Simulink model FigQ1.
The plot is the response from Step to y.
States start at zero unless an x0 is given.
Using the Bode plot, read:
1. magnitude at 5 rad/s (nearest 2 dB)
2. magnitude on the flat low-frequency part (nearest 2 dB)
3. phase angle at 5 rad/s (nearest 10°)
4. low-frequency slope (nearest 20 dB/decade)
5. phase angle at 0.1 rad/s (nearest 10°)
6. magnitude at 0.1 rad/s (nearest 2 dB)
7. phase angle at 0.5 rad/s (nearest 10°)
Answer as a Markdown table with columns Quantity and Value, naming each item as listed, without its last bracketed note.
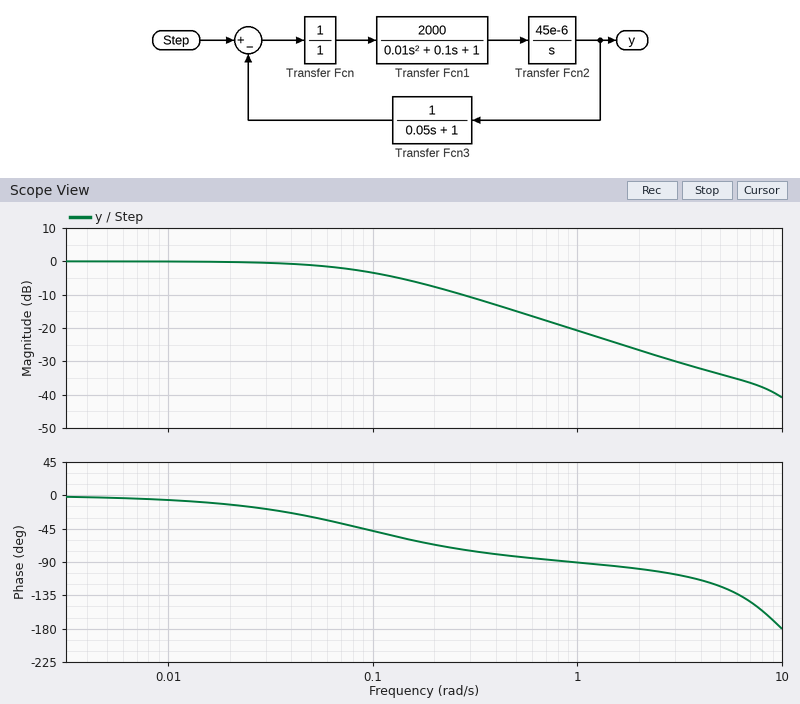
| Quantity | Value |
|---|---|
| magnitude at 5 rad/s | -34 dB |
| magnitude on the flat low-frequency part | 0 dB |
| phase angle at 5 rad/s | -120° |
| low-frequency slope | 0 dB/decade |
| phase angle at 0.1 rad/s | -50° |
| magnitude at 0.1 rad/s | -4 dB |
| phase angle at 0.5 rad/s | -80° |
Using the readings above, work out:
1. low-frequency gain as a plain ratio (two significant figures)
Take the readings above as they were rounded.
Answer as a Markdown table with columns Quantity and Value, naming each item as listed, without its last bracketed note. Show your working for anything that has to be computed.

| Quantity | Value |
|---|---|
| low-frequency gain as a plain ratio | 10^(0 / 20) = 1.0 |
